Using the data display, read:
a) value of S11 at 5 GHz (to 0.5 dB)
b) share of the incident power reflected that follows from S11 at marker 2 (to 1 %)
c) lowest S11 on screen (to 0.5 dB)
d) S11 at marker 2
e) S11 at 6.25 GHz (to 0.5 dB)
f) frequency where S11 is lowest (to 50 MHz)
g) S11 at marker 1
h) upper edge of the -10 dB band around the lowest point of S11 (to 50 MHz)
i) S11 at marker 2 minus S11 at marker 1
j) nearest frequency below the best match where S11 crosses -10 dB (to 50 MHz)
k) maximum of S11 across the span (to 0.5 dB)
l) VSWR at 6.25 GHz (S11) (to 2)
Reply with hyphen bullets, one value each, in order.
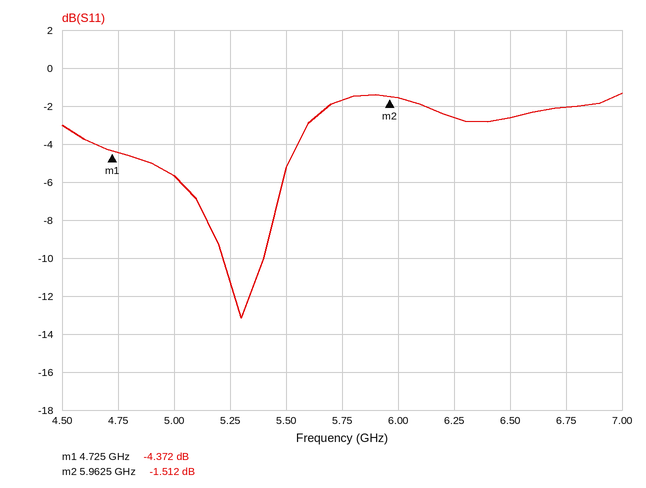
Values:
- -5.5 dB
- 71 %
- -13.0 dB
- -1.512 dB
- -2.5 dB
- 5.30 GHz
- -4.372 dB
- 5.40 GHz
- 2.860 dB
- 5.20 GHz
- -1.5 dB
- 6
